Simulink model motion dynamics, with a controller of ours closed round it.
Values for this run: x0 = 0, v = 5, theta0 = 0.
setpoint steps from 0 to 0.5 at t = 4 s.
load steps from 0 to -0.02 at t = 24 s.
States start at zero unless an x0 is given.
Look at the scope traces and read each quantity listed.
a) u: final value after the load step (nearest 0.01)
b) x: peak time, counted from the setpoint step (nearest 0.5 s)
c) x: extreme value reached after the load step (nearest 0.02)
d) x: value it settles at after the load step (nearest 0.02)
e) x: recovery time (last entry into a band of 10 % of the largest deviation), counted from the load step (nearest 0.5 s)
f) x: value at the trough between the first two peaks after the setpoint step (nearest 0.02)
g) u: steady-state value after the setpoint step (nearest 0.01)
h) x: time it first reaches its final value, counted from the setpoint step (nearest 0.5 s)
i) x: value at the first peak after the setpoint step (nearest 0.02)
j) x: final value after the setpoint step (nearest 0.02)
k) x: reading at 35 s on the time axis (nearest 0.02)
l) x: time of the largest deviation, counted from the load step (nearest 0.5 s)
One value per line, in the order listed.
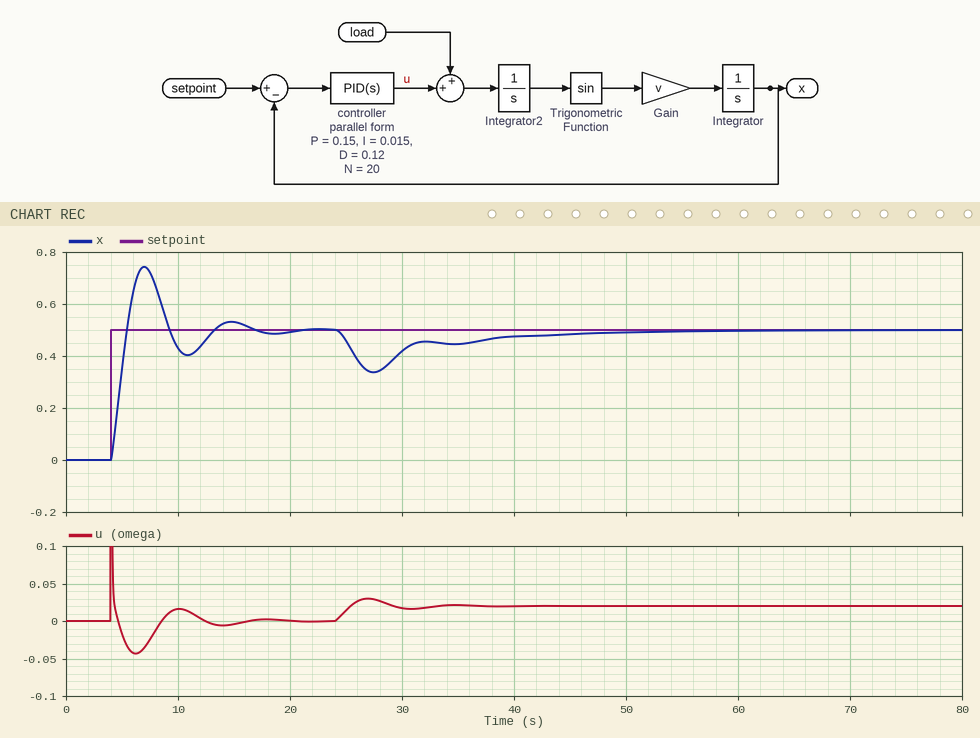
0.02
3.0 s
0.34
0.50
21.0 s
0.40
0.00
1.5 s
0.74
0.50
0.44
3.5 s
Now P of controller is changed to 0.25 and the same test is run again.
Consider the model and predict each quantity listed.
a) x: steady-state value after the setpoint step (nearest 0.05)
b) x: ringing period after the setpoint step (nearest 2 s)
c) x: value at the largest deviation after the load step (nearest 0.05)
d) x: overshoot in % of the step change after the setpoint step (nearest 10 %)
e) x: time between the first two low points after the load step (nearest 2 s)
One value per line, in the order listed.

0.50
6 s
0.40
50 %
6 s
